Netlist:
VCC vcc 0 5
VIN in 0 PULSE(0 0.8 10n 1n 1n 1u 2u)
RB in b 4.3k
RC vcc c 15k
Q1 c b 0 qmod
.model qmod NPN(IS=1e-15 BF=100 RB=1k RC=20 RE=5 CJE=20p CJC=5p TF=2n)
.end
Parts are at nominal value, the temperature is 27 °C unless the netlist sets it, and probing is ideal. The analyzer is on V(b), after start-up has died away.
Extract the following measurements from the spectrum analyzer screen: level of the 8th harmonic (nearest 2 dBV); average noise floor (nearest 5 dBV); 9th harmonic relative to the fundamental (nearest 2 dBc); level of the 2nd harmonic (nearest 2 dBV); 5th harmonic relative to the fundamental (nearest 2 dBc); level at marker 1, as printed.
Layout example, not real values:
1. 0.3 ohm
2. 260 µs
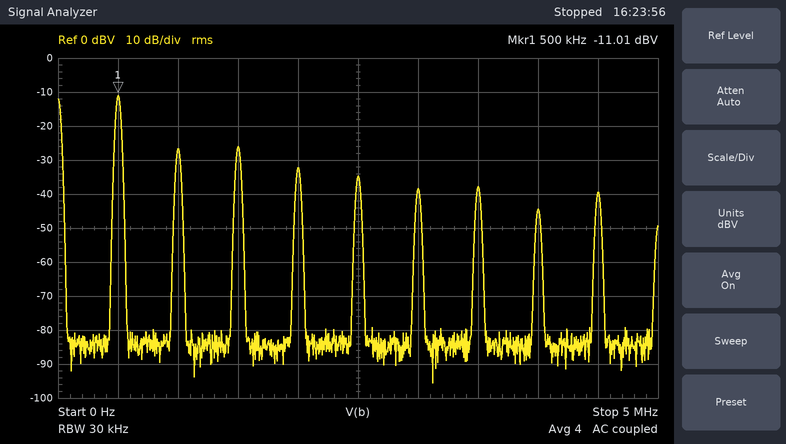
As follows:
1. -44 dBV
2. -85 dBV
3. -28 dBc
4. -26 dBV
5. -24 dBc
6. -11.01 dBV
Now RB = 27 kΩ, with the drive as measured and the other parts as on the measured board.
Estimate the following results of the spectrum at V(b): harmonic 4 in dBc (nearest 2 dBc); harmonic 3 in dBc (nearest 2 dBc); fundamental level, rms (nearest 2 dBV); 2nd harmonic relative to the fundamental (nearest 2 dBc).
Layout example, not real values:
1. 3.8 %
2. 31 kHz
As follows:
1. -36 dBc
2. -18 dBc
3. -18 dBV
4. -26 dBc
